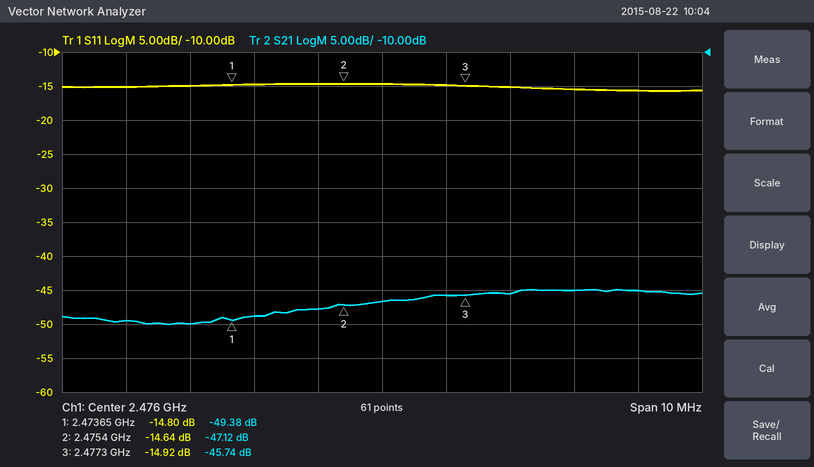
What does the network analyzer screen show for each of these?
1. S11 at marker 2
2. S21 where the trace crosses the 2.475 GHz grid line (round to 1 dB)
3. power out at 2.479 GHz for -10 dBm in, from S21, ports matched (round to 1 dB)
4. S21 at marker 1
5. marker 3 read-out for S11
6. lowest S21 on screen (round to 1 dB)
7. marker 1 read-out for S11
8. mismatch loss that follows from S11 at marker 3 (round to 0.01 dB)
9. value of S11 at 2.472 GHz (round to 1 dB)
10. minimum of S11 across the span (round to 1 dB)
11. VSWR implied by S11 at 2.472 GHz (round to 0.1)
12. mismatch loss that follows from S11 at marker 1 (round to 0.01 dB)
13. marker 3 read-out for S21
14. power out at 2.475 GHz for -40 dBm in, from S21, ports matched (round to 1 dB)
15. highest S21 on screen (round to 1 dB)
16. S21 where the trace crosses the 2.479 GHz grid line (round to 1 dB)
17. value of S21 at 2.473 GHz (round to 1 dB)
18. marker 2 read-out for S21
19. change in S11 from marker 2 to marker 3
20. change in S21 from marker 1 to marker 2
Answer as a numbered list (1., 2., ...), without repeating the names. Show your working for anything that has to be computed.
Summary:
1. -14.64 dB
2. -48 dB
3. -10 dBm + (-45 dB) = -55 dBm
4. -49.38 dB
5. -14.92 dB
6. -50 dB
7. -14.80 dB
8. −10 log10(1 − 10^(-14.92/10)) ≈ 0.14 dB
9. -15 dB
10. -16 dB
11. |Γ| = 10^(-15/20) = 0.1778; VSWR = (1 + 0.1778)/(1 − 0.1778) ≈ 1.4
12. −10 log10(1 − 10^(-14.8/10)) ≈ 0.15 dB
13. -45.74 dB
14. -40 dBm + (-48 dB) = -88 dBm
15. -45 dB
16. -45 dB
17. -50 dB
18. -47.12 dB
19. -14.92 − (-14.64) = -0.28 dB
20. -47.12 − (-49.38) = 2.26 dB
